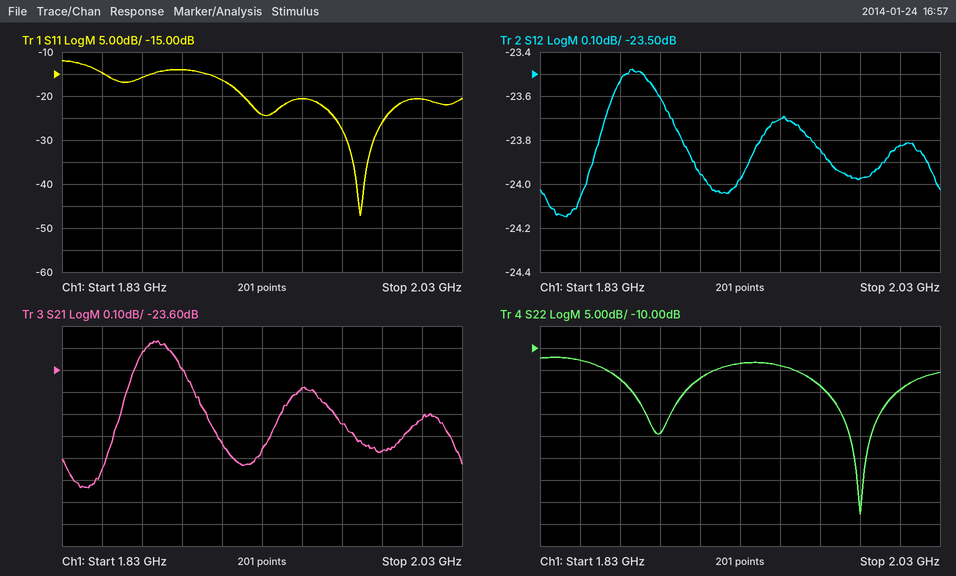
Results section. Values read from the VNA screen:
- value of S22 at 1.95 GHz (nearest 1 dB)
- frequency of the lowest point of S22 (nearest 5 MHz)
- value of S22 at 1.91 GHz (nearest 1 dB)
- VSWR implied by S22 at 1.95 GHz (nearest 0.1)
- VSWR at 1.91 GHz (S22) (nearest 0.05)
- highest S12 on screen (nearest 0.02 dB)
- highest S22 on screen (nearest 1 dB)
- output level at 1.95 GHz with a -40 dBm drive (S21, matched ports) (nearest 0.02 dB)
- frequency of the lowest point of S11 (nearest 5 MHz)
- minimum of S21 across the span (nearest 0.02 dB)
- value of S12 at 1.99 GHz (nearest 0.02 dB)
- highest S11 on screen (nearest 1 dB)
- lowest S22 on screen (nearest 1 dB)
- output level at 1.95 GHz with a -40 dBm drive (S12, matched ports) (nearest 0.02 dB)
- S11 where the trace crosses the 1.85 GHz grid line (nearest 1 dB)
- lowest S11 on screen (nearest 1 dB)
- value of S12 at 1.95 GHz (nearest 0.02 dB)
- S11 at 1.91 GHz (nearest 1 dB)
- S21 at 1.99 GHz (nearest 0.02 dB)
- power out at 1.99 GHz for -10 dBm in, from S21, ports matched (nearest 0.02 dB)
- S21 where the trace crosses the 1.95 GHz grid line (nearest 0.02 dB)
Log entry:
-14 dB
1.990 GHz
-17 dB
1.5
1.35
-23.48 dB
-12 dB
-63.68 dBm
1.980 GHz
-24.14 dB
-23.98 dB
-12 dB
-48 dB
-63.70 dBm
-15 dB
-47 dB
-23.70 dB
-16 dB
-23.96 dB
-33.96 dBm
-23.68 dB
